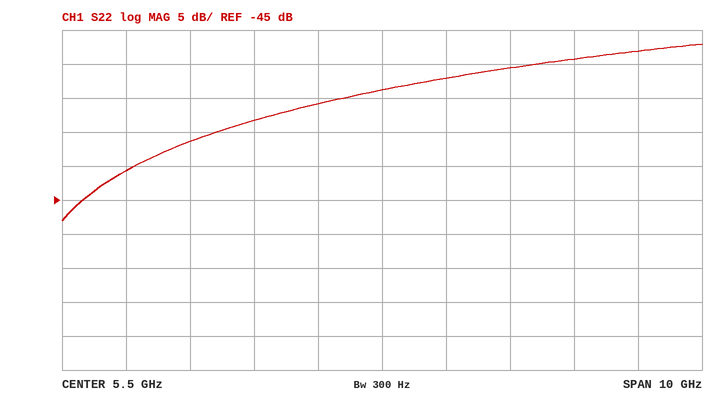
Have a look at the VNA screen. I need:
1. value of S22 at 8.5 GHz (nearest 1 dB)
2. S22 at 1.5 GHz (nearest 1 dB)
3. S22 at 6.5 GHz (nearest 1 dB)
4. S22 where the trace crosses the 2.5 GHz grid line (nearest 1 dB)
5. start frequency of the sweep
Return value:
-24 dB
-41 dB
-27 dB
-36 dB
500 MHz
